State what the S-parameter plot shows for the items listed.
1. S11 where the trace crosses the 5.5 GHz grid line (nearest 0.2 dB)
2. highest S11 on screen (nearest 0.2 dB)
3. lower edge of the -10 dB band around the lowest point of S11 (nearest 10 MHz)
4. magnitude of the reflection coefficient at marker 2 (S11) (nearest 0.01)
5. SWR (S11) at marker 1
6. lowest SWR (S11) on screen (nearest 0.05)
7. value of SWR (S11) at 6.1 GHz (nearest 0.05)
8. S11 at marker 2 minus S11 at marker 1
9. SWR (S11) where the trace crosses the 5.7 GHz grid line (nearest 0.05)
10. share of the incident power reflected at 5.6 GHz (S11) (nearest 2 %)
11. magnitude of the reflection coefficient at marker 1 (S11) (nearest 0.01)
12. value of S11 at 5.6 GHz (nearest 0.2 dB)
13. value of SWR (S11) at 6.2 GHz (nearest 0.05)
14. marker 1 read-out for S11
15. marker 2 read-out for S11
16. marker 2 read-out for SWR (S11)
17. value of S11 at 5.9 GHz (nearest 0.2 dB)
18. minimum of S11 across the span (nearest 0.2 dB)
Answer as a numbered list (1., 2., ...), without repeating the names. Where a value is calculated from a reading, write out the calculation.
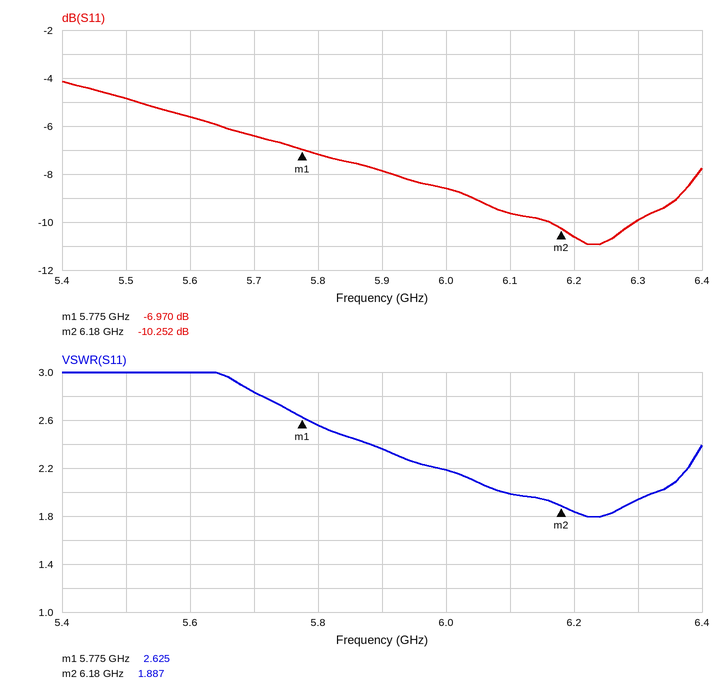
1. -4.8 dB
2. -4.2 dB
3. 6.16 GHz
4. 10^(-10.252/20) ≈ 0.31
5. 2.625
6. 1.80
7. 2.00
8. -10.252 − (-6.97) = -3.282 dB
9. 2.85
10. 10^(-5.6/10) ≈ 28 %
11. 10^(-6.97/20) ≈ 0.45
12. -5.6 dB
13. 1.85
14. -6.970 dB
15. -10.252 dB
16. 1.887
17. -7.8 dB
18. -11.0 dB
